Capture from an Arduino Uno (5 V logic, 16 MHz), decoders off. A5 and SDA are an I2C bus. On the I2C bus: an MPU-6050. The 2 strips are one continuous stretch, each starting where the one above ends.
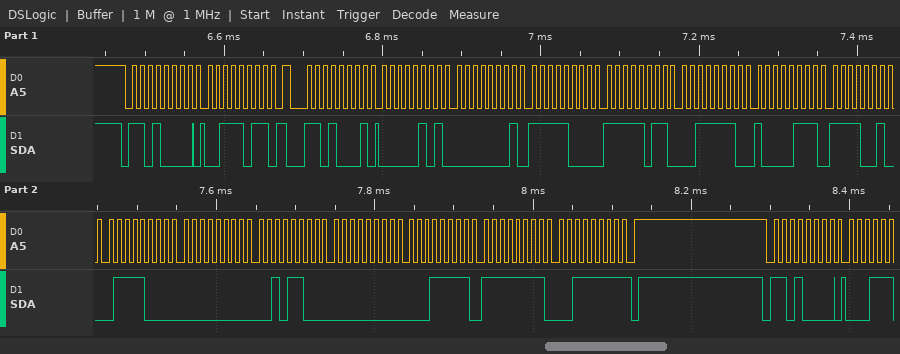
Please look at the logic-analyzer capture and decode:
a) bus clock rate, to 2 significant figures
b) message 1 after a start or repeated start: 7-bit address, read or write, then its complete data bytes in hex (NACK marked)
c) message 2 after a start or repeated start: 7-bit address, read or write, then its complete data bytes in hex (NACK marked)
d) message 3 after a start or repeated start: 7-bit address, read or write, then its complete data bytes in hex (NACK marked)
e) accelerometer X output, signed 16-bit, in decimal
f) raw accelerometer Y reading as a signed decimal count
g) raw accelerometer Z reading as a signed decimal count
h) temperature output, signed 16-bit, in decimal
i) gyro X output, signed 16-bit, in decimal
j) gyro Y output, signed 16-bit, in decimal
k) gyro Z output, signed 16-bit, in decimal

100 kHz
0x68 write: 3B
0x68 read: 05 01 F8 FB 3E 87 F2 78 00 2C 00 1F FF 3F NACK
0x68 write
1281
-1797
16007
-3464
44
31
-193
